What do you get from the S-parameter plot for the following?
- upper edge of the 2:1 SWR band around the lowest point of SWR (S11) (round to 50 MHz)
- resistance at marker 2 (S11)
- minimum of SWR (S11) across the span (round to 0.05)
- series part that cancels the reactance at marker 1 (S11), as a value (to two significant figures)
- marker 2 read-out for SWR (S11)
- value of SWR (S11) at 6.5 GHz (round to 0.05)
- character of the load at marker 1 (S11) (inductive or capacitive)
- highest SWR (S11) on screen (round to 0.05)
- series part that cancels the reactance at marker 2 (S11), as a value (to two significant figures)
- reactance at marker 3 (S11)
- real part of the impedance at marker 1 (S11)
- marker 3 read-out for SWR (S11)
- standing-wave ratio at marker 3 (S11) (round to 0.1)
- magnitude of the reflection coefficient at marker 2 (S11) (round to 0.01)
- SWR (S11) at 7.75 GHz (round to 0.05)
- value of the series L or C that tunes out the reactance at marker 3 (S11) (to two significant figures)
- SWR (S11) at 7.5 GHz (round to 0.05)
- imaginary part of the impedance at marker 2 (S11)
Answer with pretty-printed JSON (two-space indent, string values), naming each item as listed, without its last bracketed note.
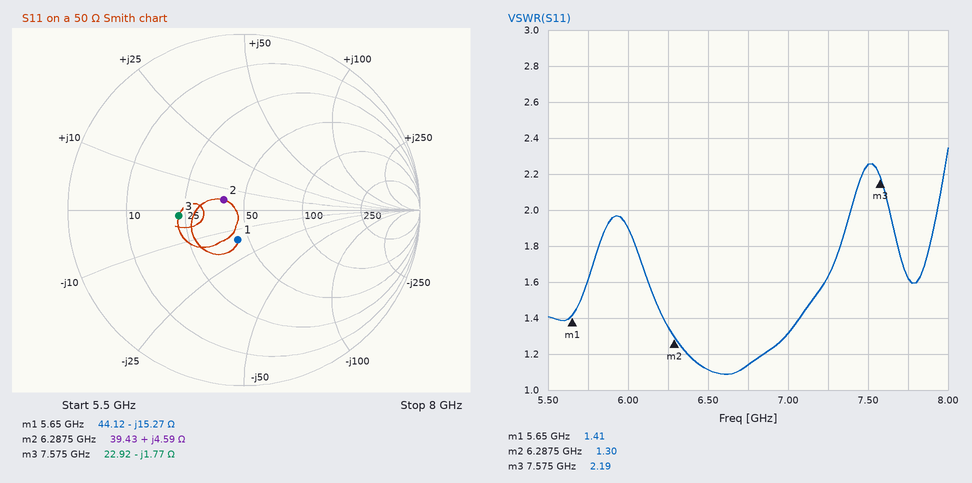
{
  "upper edge of the 2:1 SWR band around the lowest point of SWR (S11)": "7.40 GHz",
  "resistance at marker 2": "39.43 Ω",
  "minimum of SWR (S11) across the span": "1.10",
  "series part that cancels the reactance at marker 1 (S11), as a value": "430 pH",
  "marker 2 read-out for SWR": "1.30",
  "value of SWR (S11) at 6.5 GHz": "1.10",
  "character of the load at marker 1 (S11)": "capacitive",
  "highest SWR (S11) on screen": "2.35",
  "series part that cancels the reactance at marker 2 (S11), as a value": "5.5 pF",
  "reactance at marker 3": "-1.77 Ω",
  "real part of the impedance at marker 1": "44.12 Ω",
  "marker 3 read-out for SWR": "2.19",
  "standing-wave ratio at marker 3 (S11)": "2.2",
  "magnitude of the reflection coefficient at marker 2 (S11)": "0.13",
  "SWR (S11) at 7.75 GHz": "1.60",
  "value of the series L or C that tunes out the reactance at marker 3 (S11)": "37 pH",
  "SWR (S11) at 7.5 GHz": "2.25",
  "imaginary part of the impedance at marker 2": "+4.59 Ω"
}
